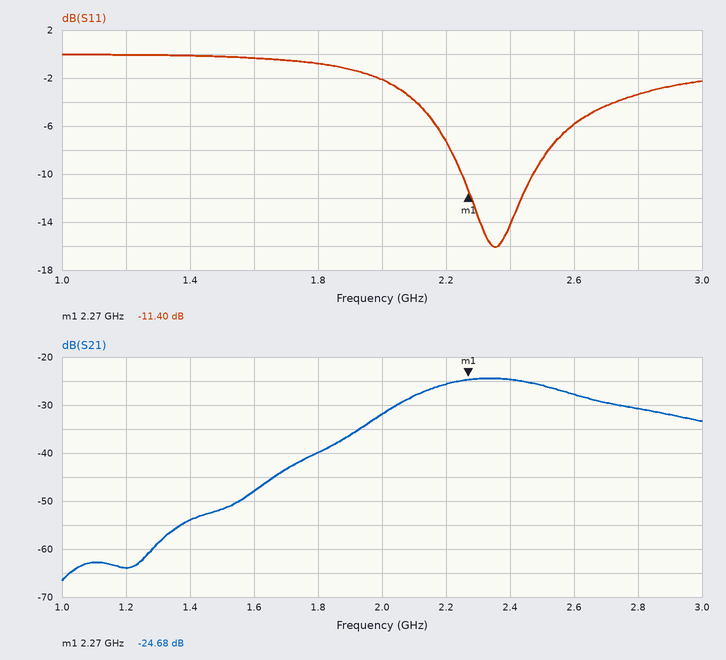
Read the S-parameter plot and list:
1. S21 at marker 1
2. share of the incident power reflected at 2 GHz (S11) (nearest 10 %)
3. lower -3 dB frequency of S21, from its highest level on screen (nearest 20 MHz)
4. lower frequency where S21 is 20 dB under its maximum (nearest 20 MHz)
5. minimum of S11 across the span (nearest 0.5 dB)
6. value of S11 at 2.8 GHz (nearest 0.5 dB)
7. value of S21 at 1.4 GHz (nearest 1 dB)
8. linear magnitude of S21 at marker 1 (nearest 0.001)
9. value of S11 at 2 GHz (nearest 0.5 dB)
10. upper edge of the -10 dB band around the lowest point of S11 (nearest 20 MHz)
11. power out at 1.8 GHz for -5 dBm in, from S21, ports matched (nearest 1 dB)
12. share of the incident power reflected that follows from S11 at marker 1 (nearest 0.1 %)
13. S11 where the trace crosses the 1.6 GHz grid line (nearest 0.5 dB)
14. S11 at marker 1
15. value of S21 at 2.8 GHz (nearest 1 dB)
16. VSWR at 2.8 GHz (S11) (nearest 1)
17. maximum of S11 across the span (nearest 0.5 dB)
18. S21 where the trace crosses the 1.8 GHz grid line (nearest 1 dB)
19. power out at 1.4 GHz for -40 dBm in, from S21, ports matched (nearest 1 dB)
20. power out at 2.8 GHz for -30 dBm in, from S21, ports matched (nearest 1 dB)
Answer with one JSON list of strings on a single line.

["-24.68 dB", "60 %", "2.12 GHz", "1.68 GHz", "-16.0 dB", "-3.5 dB", "-54 dB", "0.058", "-2.0 dB", "2.48 GHz", "-45 dBm", "7.2 %", "-0.5 dB", "-11.40 dB", "-31 dB", "5", "0.0 dB", "-40 dB", "-94 dBm", "-61 dBm"]
